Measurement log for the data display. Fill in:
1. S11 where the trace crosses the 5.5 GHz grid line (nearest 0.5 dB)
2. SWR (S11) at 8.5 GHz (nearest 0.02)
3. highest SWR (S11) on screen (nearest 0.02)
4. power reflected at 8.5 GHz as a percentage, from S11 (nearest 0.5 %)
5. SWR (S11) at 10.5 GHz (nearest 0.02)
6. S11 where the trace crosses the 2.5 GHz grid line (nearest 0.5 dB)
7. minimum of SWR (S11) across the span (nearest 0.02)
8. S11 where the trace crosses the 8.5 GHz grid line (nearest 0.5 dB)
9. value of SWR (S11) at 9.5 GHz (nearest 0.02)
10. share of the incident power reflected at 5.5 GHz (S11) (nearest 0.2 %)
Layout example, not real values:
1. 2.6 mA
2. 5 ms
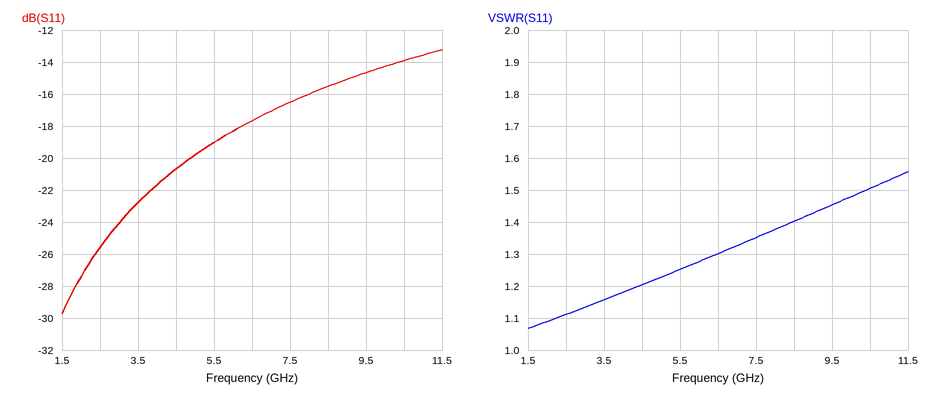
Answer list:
1. -19.0 dB
2. 1.40
3. 1.56
4. 3.0 %
5. 1.50
6. -25.5 dB
7. 1.06
8. -15.5 dB
9. 1.46
10. 1.2 %
